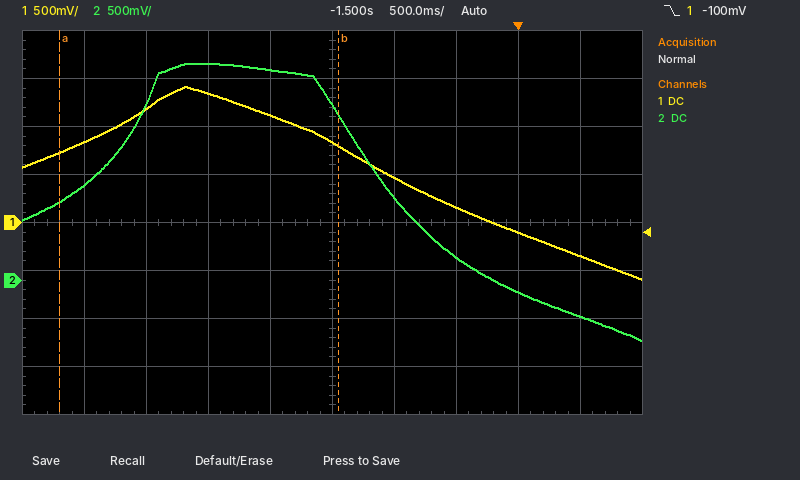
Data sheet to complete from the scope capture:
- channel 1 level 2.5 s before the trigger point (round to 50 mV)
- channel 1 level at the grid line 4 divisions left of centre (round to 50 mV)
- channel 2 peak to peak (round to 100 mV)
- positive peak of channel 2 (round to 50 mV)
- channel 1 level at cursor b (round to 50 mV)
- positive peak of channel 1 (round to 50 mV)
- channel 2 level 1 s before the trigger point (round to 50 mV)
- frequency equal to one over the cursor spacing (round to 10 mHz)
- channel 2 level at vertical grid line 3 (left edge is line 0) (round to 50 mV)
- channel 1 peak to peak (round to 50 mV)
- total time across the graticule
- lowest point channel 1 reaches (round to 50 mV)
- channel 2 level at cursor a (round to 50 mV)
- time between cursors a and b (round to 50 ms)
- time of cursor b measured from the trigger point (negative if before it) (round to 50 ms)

1.35 V
850 mV
2.90 V
2.25 V
800 mV
1.40 V
850 mV
440 mHz
2.25 V
2.00 V
5 s
-600 mV
800 mV
2.25 s
-1.45 s
